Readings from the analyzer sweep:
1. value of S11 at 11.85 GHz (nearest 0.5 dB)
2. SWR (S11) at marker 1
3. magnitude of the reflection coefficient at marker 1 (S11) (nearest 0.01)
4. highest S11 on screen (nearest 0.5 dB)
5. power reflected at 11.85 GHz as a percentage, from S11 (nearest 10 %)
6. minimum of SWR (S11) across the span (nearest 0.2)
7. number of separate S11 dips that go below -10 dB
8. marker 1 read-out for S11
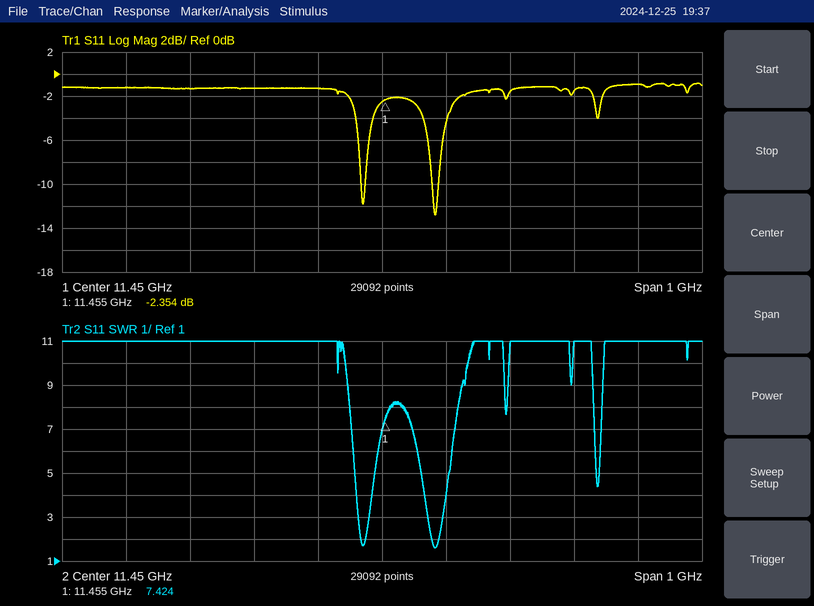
-1.0 dB
7.424
0.76
-1.0 dB
80 %
1.6
2
-2.354 dB
